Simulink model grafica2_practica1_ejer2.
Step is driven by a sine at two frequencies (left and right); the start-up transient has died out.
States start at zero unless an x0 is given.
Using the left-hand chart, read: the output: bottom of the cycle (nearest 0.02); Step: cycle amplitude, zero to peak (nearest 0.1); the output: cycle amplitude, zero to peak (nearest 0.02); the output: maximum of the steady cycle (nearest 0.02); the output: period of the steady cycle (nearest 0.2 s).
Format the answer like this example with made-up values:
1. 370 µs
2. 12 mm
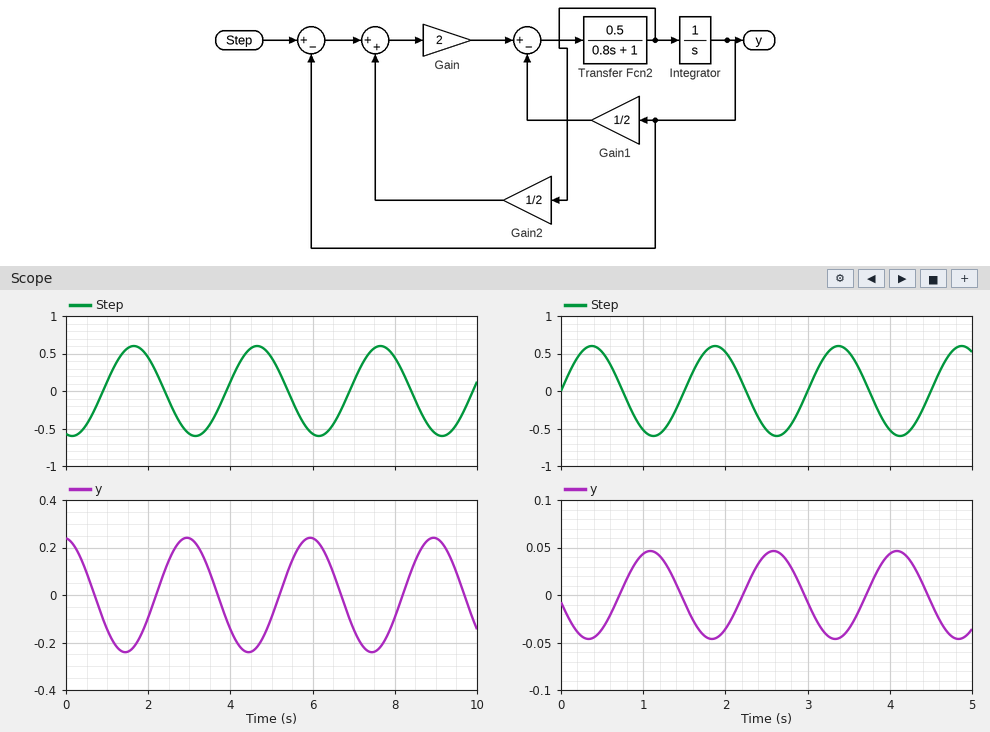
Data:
1. -0.24
2. 0.6
3. 0.24
4. 0.24
5. 3.0 s
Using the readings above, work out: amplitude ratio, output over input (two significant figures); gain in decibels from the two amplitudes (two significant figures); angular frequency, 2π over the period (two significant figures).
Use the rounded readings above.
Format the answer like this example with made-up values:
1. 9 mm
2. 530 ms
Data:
1. 0.40
2. -8.0 dB
3. 2.1 rad/s
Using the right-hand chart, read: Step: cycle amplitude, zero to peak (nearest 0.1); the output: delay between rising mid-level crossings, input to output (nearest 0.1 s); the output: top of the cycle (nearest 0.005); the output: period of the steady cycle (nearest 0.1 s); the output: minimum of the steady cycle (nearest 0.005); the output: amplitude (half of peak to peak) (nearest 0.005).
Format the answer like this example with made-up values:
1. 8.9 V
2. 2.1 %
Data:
1. 0.6
2. 0.7 s
3. 0.045
4. 1.5 s
5. -0.045
6. 0.045
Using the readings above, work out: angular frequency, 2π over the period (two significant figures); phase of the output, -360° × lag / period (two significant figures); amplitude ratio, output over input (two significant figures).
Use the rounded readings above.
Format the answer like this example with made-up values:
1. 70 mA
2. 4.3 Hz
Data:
1. 4.2 rad/s
2. -170°
3. 0.075
